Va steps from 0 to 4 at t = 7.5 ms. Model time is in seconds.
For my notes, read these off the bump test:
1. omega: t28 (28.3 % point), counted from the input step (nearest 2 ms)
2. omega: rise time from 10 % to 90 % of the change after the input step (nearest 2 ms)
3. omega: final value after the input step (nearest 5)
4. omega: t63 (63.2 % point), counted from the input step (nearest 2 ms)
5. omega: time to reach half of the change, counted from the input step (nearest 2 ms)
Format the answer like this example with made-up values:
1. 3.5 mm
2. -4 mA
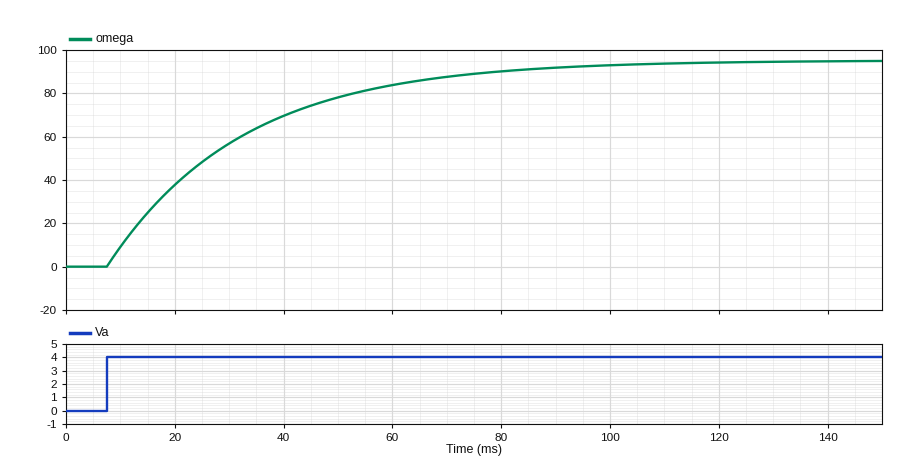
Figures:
1. 8 ms
2. 54 ms
3. 95
4. 24 ms
5. 18 ms
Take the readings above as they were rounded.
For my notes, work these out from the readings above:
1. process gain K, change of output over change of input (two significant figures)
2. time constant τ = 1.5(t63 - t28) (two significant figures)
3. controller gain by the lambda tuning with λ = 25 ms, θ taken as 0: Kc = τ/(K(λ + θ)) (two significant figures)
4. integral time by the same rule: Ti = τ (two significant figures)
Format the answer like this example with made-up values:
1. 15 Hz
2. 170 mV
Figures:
1. 24
2. 24 ms
3. 0.040
4. 24 ms
